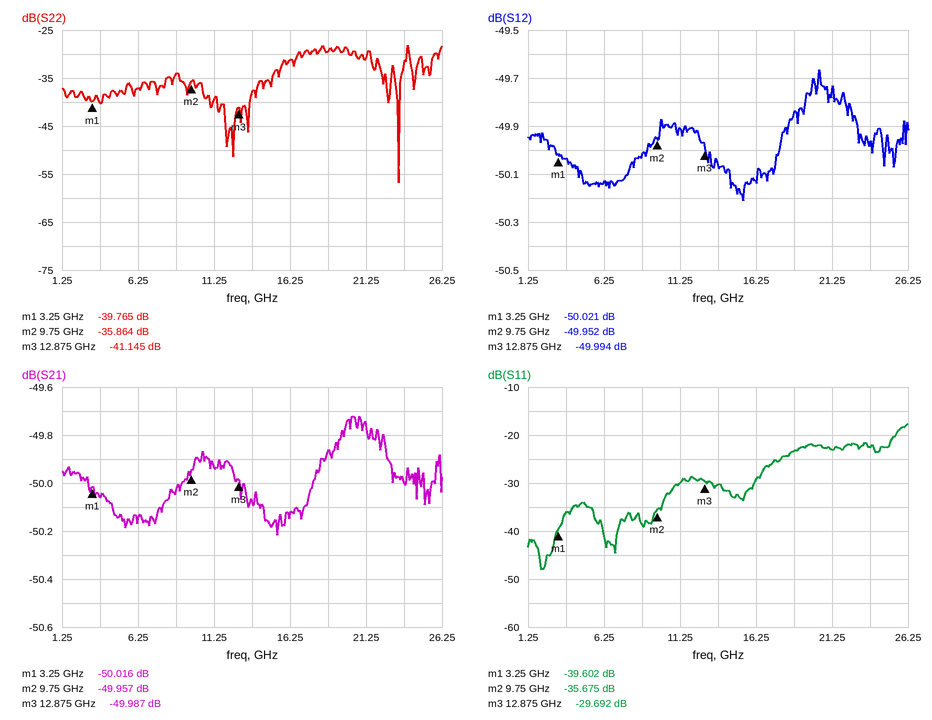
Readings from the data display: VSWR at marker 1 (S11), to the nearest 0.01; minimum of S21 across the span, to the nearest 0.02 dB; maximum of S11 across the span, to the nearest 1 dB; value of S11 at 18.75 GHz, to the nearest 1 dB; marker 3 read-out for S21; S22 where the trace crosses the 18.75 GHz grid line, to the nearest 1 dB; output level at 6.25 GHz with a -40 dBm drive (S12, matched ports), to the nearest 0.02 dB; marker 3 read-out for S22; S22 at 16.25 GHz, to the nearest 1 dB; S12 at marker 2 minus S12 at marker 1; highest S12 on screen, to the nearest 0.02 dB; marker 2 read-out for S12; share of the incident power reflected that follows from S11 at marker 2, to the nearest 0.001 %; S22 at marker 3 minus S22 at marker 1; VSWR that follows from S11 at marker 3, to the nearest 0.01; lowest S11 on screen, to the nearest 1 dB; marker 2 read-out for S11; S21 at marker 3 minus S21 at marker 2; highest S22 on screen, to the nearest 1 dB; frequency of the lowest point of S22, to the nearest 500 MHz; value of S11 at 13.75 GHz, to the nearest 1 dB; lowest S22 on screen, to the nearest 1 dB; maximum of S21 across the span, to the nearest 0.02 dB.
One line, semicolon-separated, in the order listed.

1.02; -50.22 dB; -18 dB; -23 dB; -49.987 dB; -29 dB; -90.14 dBm; -41.145 dB; -31 dB; 0.069 dB; -49.66 dB; -49.952 dB; 0.027 %; -1.380 dB; 1.07; -48 dB; -35.675 dB; -0.030 dB; -28 dB; 23.5 GHz; -30 dB; -57 dB; -49.72 dB
